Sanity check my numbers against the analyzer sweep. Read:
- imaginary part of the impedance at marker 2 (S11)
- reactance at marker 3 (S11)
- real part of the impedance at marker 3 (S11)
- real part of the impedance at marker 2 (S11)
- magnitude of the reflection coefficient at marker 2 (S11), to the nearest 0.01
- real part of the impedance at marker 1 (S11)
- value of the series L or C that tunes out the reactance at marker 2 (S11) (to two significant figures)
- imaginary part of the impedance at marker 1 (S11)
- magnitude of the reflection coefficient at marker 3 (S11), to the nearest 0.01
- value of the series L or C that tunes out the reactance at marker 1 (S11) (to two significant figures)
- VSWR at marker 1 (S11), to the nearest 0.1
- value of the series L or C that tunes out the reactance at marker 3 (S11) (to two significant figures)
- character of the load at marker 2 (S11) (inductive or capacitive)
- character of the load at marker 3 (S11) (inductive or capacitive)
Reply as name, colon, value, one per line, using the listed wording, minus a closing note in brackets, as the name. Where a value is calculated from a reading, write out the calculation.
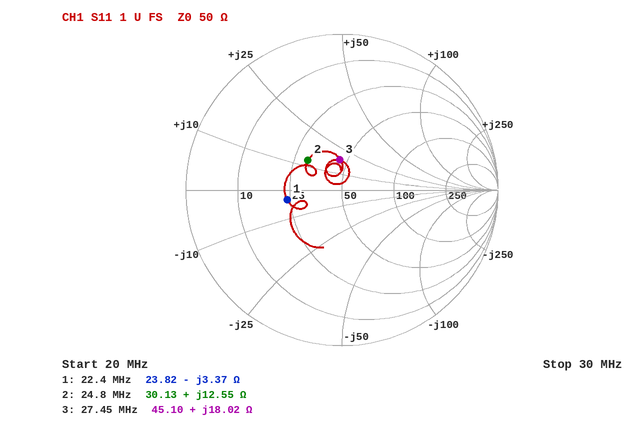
imaginary part of the impedance at marker 2: +12.55 Ω
reactance at marker 3: +18.02 Ω
real part of the impedance at marker 3: 45.10 Ω
real part of the impedance at marker 2: 30.13 Ω
magnitude of the reflection coefficient at marker 2 (S11), to the nearest 0.01: 0.29
real part of the impedance at marker 1: 23.82 Ω
value of the series L or C that tunes out the reactance at marker 2 (S11): C = 1/(2π × 24.8 MHz × 12.55 Ω) ≈ 511 pF, so 510 pF to two significant figures
imaginary part of the impedance at marker 1: -3.37 Ω
magnitude of the reflection coefficient at marker 3 (S11), to the nearest 0.01: 0.19
value of the series L or C that tunes out the reactance at marker 1 (S11): L = 3.37 Ω/(2π × 22.4 MHz) ≈ 24 nH
VSWR at marker 1 (S11), to the nearest 0.1: 2.1
value of the series L or C that tunes out the reactance at marker 3 (S11): C = 1/(2π × 27.45 MHz × 18.02 Ω) ≈ 322 pF, so 320 pF to two significant figures
character of the load at marker 2 (S11): inductive
character of the load at marker 3 (S11): inductive
